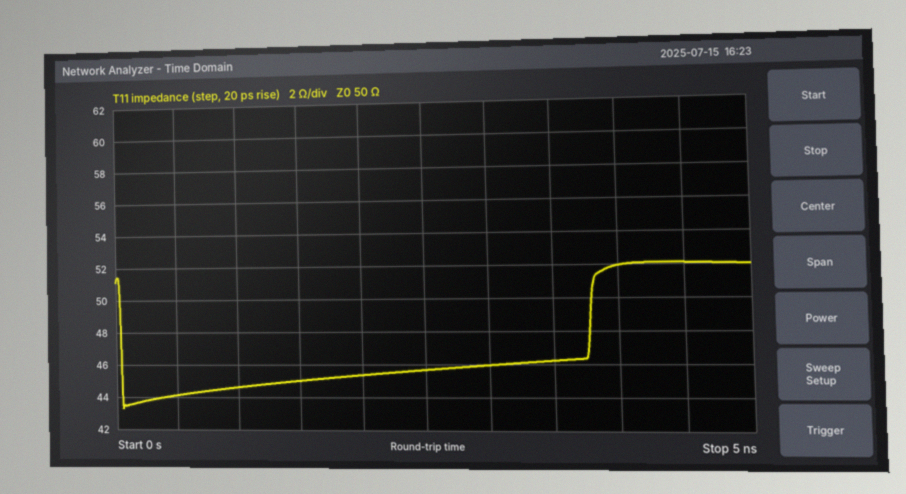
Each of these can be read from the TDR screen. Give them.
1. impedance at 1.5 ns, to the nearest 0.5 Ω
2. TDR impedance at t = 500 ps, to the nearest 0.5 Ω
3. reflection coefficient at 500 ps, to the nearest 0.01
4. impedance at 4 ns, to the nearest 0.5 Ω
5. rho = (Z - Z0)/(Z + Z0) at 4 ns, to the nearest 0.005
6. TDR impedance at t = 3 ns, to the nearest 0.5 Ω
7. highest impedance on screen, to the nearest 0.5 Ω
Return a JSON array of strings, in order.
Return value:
["45.0 Ω", "44.0 Ω", "-0.06", "52.0 Ω", "+0.020", "46.0 Ω", "52.0 Ω"]
